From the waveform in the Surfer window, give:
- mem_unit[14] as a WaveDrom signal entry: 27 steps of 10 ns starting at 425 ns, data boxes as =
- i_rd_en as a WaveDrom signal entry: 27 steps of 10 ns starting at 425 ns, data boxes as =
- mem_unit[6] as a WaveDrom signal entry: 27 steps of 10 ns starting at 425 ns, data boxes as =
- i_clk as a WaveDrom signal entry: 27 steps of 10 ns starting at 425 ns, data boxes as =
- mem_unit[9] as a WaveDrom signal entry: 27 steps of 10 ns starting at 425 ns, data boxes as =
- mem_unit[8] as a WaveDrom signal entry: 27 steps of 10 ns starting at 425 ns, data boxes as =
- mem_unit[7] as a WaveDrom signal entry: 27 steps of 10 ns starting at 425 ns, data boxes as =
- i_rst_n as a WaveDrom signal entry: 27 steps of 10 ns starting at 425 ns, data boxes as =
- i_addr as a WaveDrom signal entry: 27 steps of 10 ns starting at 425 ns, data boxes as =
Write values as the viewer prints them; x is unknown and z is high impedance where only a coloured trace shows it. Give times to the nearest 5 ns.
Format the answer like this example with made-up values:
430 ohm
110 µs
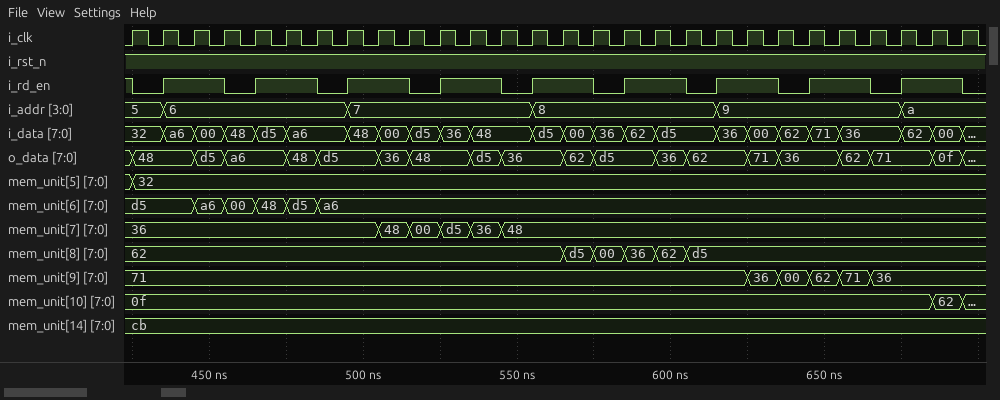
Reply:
{name: 'mem_unit[14]', wave: '=..........................', data: 'cb'}
{name: 'i_rd_en', wave: '01.01.01.01.01.01.01.01.01.'}
{name: 'mem_unit[6]', wave: '=.=====....................', data: 'd5 a6 00 48 d5 a6'}
{name: 'i_clk', wave: 'p..........................'}
{name: 'mem_unit[9]', wave: '=...................=====..', data: '71 36 00 62 71 36'}
{name: 'mem_unit[8]', wave: '=.............=====........', data: '62 d5 00 36 62 d5'}
{name: 'mem_unit[7]', wave: '=.......=====..............', data: '36 48 00 d5 36 48'}
{name: 'i_rst_n', wave: '1..........................'}
{name: 'i_addr', wave: '==.....=.....=.....=.....=.', data: '5 6 7 8 9 a'}
